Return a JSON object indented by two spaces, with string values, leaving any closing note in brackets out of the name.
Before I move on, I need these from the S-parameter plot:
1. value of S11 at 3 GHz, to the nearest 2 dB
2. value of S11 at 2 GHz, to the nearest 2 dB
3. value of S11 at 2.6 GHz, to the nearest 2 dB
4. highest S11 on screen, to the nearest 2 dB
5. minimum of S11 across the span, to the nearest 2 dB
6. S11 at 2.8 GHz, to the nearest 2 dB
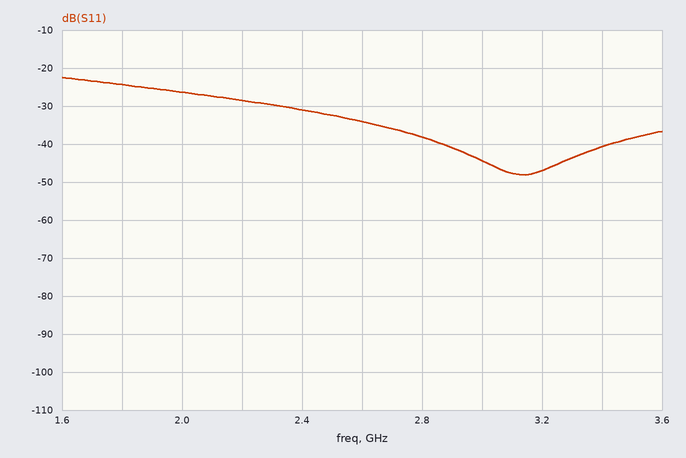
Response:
{
  "value of S11 at 3 GHz, to the nearest 2 dB": "-44 dB",
  "value of S11 at 2 GHz, to the nearest 2 dB": "-26 dB",
  "value of S11 at 2.6 GHz, to the nearest 2 dB": "-34 dB",
  "highest S11 on screen, to the nearest 2 dB": "-22 dB",
  "minimum of S11 across the span, to the nearest 2 dB": "-48 dB",
  "S11 at 2.8 GHz, to the nearest 2 dB": "-38 dB"
}
